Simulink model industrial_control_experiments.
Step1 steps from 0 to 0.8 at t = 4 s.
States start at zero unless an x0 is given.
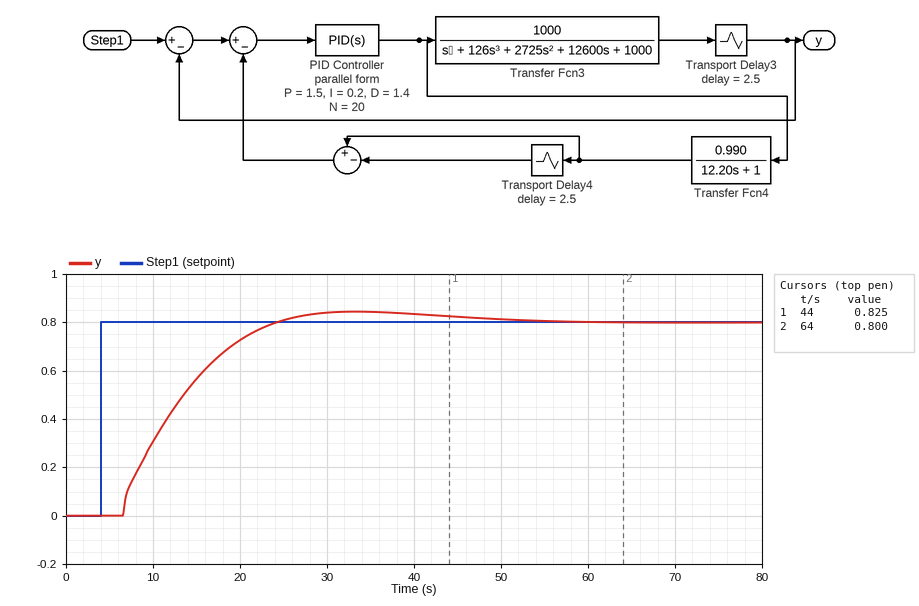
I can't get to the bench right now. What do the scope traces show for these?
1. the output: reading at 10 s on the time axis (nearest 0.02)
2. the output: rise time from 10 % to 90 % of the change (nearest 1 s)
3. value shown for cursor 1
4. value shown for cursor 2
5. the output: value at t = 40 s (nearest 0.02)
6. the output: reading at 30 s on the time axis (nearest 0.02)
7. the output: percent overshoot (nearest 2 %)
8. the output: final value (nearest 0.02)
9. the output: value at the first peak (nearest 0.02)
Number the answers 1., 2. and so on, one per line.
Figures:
1. 0.30
2. 13 s
3. 0.825
4. 0.800
5. 0.84
6. 0.84
7. 6 %
8. 0.80
9. 0.84
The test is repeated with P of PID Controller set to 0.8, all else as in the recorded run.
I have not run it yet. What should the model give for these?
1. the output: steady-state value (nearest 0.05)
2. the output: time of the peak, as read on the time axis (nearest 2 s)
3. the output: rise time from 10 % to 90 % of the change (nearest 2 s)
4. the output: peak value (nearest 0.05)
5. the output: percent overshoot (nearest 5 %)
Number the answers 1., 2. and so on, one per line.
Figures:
1. 0.80
2. 34 s
3. 14 s
4. 0.90
5. 15 %
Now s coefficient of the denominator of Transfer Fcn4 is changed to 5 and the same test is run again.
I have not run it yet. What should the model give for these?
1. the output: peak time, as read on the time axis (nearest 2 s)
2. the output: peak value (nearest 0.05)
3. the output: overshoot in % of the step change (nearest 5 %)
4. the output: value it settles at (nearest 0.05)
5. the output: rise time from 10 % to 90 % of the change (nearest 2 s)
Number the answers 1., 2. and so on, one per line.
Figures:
1. 34 s
2. 0.90
3. 10 %
4. 0.80
5. 14 s
